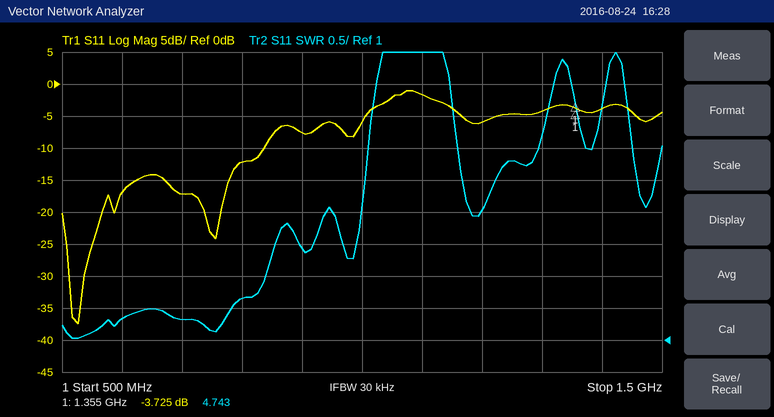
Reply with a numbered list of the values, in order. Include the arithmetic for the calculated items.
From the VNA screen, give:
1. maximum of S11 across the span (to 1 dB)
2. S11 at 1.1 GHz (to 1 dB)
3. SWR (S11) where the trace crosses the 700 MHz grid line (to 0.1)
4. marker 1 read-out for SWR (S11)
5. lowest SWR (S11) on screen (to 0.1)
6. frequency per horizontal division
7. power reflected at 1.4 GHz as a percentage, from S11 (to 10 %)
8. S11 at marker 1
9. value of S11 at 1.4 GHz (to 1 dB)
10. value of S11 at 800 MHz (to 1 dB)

1. -1 dB
2. -2 dB
3. 1.3
4. 4.743
5. 1.0
6. 100 MHz
7. 10^(-4/10) ≈ 40 %
8. -3.725 dB
9. -4 dB
10. -12 dB
